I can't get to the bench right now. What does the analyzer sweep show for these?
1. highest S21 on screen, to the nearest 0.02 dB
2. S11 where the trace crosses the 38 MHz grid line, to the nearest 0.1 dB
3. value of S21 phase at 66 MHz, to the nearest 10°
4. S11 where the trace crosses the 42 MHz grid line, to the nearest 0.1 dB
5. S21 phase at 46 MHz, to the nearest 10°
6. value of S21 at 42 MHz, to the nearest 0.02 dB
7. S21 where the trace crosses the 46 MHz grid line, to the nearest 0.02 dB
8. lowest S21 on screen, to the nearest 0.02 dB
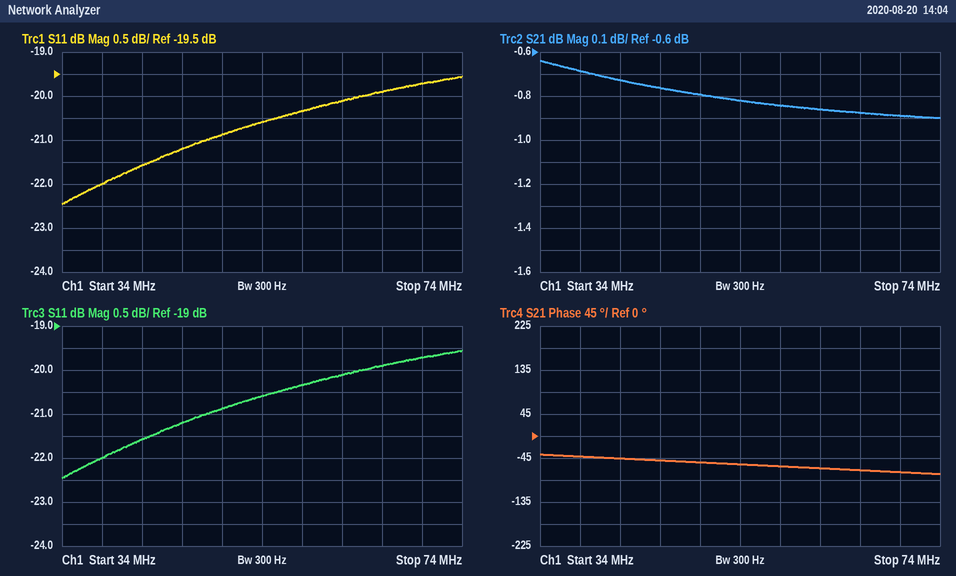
-0.64 dB
-22.0 dB
-70°
-21.6 dB
-50°
-0.72 dB
-0.76 dB
-0.90 dB
